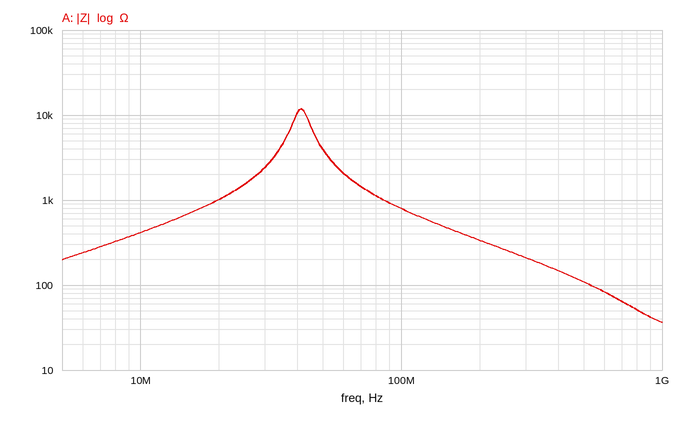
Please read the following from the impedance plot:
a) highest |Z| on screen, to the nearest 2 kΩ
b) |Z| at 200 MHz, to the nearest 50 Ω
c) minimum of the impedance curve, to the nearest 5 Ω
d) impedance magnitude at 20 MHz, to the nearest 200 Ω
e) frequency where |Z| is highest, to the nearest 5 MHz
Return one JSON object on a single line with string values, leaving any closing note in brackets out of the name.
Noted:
{"highest |Z| on screen, to the nearest 2 kΩ": "12 kΩ", "|Z| at 200 MHz, to the nearest 50 Ω": "350 Ω", "minimum of the impedance curve, to the nearest 5 Ω": "35 Ω", "impedance magnitude at 20 MHz, to the nearest 200 Ω": "1.0 kΩ", "frequency where |Z| is highest, to the nearest 5 MHz": "40 MHz"}
